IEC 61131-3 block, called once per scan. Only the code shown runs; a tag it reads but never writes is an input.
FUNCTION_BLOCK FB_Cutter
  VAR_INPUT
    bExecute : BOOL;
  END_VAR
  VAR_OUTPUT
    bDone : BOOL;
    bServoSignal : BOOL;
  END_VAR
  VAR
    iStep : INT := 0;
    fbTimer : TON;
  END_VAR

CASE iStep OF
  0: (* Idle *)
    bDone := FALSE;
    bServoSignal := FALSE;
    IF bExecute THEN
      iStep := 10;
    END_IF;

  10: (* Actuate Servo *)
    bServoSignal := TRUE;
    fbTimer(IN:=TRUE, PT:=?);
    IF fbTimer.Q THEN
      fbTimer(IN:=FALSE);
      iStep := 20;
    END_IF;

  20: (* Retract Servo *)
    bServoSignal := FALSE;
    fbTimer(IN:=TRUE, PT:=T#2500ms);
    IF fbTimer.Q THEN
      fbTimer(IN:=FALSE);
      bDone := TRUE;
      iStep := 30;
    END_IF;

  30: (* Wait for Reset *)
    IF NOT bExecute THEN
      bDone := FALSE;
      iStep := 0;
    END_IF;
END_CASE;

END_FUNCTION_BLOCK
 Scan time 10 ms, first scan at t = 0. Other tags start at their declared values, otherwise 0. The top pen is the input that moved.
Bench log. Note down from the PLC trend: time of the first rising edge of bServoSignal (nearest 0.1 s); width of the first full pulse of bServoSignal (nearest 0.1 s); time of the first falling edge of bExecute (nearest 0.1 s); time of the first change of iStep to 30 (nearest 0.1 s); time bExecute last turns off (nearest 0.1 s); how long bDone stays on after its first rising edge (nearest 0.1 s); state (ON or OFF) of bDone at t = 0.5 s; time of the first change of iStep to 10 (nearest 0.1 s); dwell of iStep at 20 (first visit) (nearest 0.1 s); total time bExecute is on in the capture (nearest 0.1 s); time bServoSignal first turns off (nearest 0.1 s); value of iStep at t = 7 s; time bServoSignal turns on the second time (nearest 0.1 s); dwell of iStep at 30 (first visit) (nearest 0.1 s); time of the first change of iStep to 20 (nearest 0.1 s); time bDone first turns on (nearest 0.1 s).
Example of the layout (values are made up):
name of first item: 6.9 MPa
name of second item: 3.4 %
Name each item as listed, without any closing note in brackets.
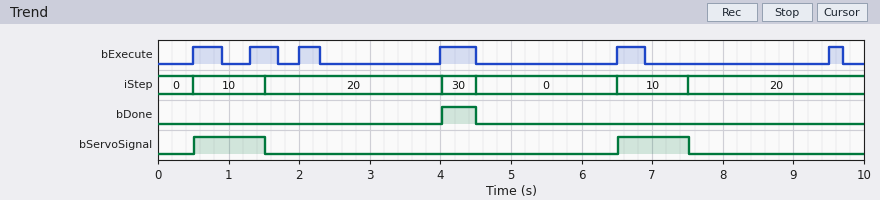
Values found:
time of the first rising edge of bServoSignal: 0.5 s
width of the first full pulse of bServoSignal: 1.0 s
time of the first falling edge of bExecute: 0.9 s
time of the first change of iStep to 30: 4.0 s
time bExecute last turns off: 9.7 s
how long bDone stays on after its first rising edge: 0.5 s
state (ON or OFF) of bDone at t = 0.5 s: OFF
time of the first change of iStep to 10: 0.5 s
dwell of iStep at 20 (first visit): 2.5 s
total time bExecute is on in the capture: 2.2 s
time bServoSignal first turns off: 1.5 s
value of iStep at t = 7 s: 10
time bServoSignal turns on the second time: 6.5 s
dwell of iStep at 30 (first visit): 0.5 s
time of the first change of iStep to 20: 1.5 s
time bDone first turns on: 4.0 s
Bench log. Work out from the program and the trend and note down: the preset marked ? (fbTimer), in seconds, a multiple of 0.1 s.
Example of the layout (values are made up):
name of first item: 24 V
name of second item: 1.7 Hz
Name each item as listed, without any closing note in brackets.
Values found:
the preset marked ? (fbTimer), in seconds, a multiple of 0.1 s: 1.0 s
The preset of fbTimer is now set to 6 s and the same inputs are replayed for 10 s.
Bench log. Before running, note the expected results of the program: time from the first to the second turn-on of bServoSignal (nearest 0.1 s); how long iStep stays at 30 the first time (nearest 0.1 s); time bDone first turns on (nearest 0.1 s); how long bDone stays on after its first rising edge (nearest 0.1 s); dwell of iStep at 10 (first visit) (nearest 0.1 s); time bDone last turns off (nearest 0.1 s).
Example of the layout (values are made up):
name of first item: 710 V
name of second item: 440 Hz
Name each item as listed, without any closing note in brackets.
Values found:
time from the first to the second turn-on of bServoSignal: 9.0 s
how long iStep stays at 30 the first time: 0.0 s
time bDone first turns on: 9.0 s
how long bDone stays on after its first rising edge: 0.0 s
dwell of iStep at 10 (first visit): 6.0 s
time bDone last turns off: 9.0 s
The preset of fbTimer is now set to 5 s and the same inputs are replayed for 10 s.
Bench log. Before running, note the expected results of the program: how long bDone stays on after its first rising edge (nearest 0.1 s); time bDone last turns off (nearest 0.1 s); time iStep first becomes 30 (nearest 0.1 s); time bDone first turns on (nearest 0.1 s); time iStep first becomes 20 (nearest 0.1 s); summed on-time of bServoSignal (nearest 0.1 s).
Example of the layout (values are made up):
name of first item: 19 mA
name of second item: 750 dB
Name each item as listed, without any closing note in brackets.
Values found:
how long bDone stays on after its first rising edge: 0.0 s
time bDone last turns off: 8.0 s
time iStep first becomes 30: 8.0 s
time bDone first turns on: 8.0 s
time iStep first becomes 20: 5.5 s
summed on-time of bServoSignal: 5.5 s
